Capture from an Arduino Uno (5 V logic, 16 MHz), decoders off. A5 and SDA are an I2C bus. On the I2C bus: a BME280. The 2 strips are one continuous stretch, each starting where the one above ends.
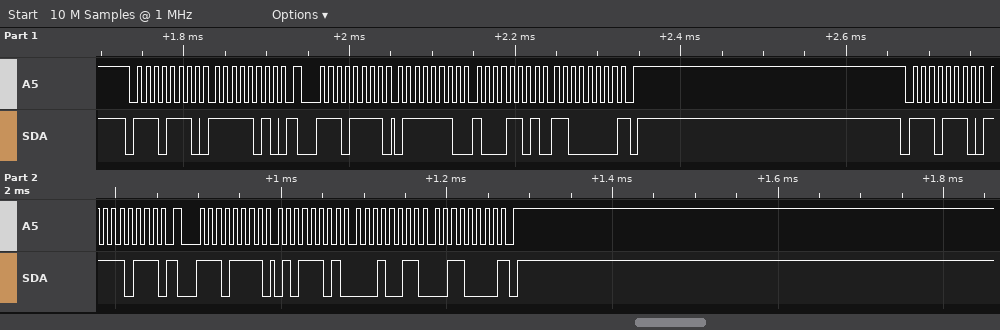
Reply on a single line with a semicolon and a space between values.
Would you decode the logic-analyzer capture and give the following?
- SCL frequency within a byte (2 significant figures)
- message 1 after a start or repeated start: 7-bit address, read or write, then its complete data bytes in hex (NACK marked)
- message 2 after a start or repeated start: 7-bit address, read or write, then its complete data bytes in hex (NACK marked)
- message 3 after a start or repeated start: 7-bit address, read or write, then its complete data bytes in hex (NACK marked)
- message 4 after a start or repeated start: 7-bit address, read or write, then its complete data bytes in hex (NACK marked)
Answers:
100 kHz; 0x77 write: FA; 0x77 read: 7E 8D C0 NACK; 0x77 write: F7; 0x77 read: 5D 13 30 NACK
